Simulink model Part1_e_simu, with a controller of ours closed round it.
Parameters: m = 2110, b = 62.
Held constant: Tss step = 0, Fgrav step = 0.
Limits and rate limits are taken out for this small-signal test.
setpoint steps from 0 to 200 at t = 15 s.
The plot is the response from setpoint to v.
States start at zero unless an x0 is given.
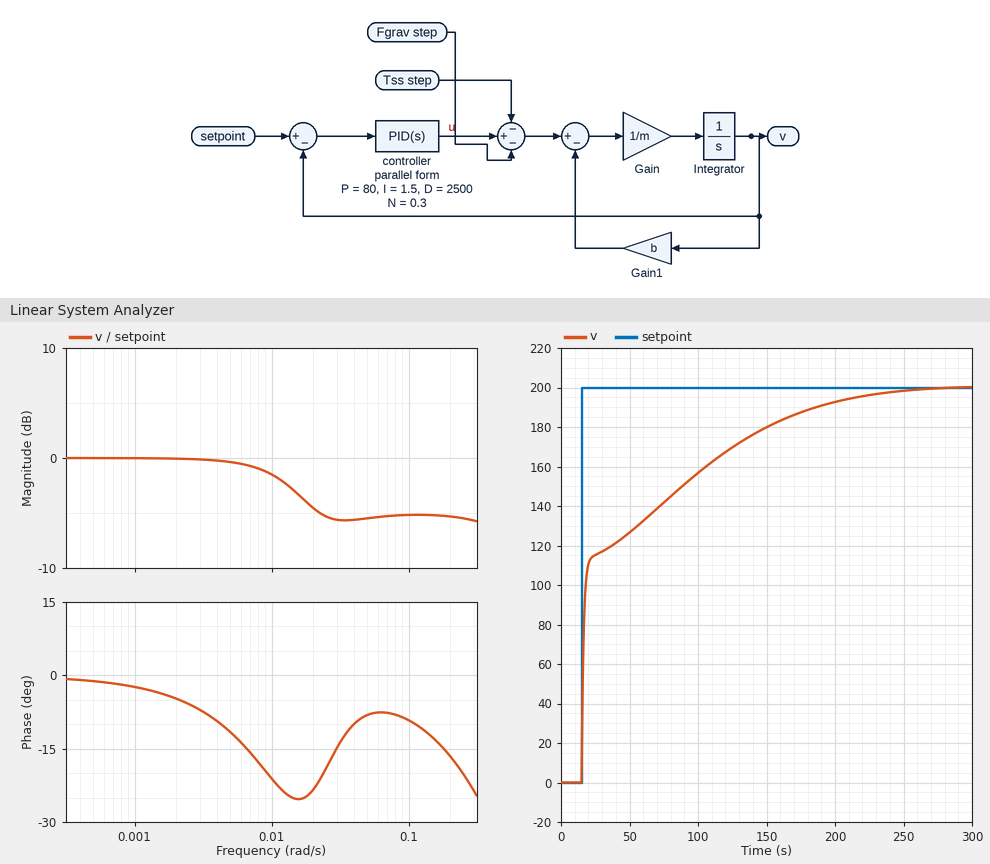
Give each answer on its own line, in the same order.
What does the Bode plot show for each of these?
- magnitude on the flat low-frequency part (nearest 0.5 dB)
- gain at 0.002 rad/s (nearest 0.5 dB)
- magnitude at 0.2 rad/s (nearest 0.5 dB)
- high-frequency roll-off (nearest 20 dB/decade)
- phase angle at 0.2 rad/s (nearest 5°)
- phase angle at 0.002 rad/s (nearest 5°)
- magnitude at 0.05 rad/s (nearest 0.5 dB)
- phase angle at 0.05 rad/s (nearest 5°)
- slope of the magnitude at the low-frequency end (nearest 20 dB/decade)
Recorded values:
0.0 dB
0.0 dB
-5.5 dB
0 dB/decade
-15°
-5°
-5.5 dB
-10°
0 dB/decade
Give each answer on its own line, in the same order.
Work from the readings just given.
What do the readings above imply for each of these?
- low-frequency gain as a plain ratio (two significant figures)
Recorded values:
1.0
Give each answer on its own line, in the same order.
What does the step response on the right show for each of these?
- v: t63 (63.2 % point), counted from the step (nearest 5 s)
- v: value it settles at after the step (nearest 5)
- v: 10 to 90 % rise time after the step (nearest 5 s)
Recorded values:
35 s
200
135 s
